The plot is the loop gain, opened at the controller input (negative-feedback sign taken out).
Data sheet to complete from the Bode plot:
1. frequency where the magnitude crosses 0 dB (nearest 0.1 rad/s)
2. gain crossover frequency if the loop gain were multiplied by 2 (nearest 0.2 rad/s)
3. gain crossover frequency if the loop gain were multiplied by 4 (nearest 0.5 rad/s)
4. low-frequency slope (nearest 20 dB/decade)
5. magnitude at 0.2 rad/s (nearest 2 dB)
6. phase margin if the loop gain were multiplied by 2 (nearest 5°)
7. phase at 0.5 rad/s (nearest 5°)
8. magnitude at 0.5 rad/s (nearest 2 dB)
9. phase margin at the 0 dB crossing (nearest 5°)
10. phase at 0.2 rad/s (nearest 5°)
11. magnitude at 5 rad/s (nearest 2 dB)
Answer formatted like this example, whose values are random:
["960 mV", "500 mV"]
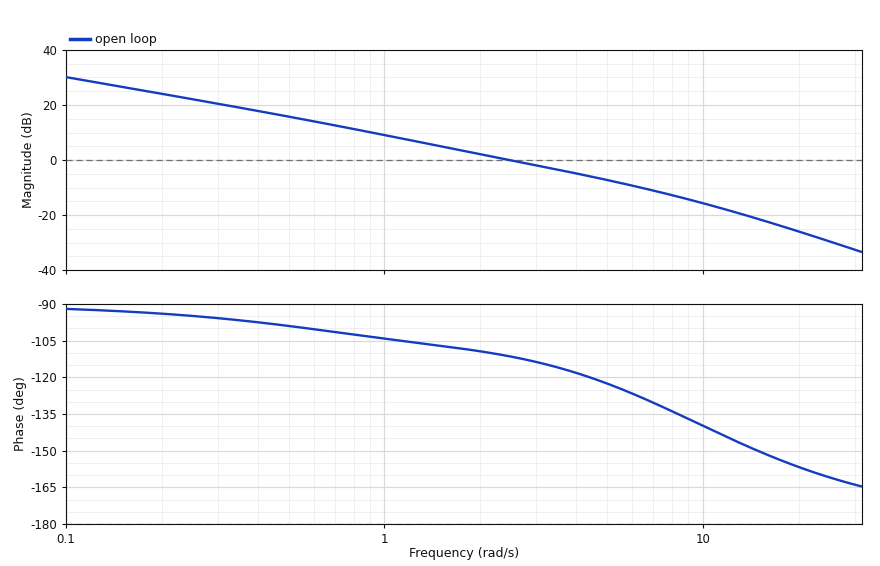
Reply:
["2.5 rad/s", "4.4 rad/s", "7.5 rad/s", "-20 dB/decade", "24 dB", "60°", "-100°", "16 dB", "70°", "-95°", "-8 dB"]
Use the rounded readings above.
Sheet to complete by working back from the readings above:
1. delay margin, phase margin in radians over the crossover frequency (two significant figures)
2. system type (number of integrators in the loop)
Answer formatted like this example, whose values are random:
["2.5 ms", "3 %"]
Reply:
["0.49 s", "1"]
